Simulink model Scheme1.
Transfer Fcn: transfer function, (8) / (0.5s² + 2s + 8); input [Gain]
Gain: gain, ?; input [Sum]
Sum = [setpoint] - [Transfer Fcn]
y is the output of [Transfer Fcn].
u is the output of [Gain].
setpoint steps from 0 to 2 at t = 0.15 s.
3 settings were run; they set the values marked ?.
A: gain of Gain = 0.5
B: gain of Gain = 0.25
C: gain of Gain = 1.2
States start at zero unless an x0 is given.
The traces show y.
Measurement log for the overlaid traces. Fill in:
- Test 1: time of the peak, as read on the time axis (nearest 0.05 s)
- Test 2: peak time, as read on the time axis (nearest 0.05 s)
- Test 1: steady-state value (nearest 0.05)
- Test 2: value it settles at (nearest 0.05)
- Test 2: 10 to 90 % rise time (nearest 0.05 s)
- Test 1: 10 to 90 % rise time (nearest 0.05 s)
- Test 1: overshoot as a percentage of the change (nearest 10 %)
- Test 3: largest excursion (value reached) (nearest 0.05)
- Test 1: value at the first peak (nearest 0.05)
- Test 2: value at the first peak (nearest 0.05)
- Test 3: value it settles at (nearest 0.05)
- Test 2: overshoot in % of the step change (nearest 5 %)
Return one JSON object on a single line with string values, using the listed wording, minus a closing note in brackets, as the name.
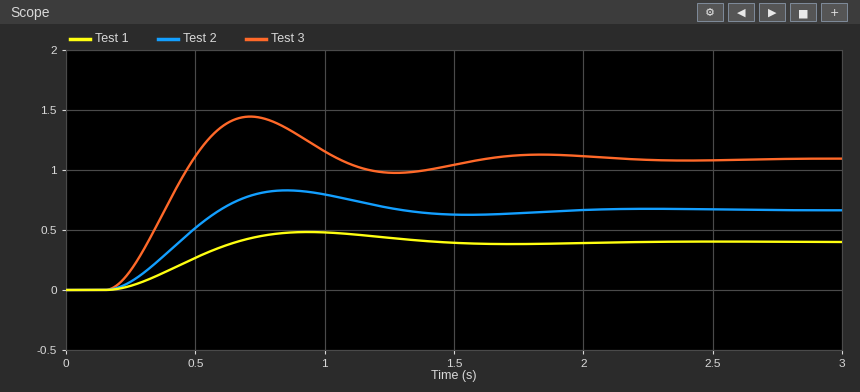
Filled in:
{"Test 1: time of the peak, as read on the time axis": "0.95 s", "Test 2: peak time, as read on the time axis": "0.85 s", "Test 1: steady-state value": "0.40", "Test 2: value it settles at": "0.65", "Test 2: 10 to 90 % rise time": "0.30 s", "Test 1: 10 to 90 % rise time": "0.35 s", "Test 1: overshoot as a percentage of the change": "20 %", "Test 3: largest excursion (value reached)": "1.45", "Test 1: value at the first peak": "0.50", "Test 2: value at the first peak": "0.85", "Test 3: value it settles at": "1.10", "Test 2: overshoot in % of the step change": "25 %"}
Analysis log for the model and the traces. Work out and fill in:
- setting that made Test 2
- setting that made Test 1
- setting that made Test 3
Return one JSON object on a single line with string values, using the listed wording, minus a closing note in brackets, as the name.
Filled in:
{"setting that made Test 2": "A", "setting that made Test 1": "B", "setting that made Test 3": "C"}
